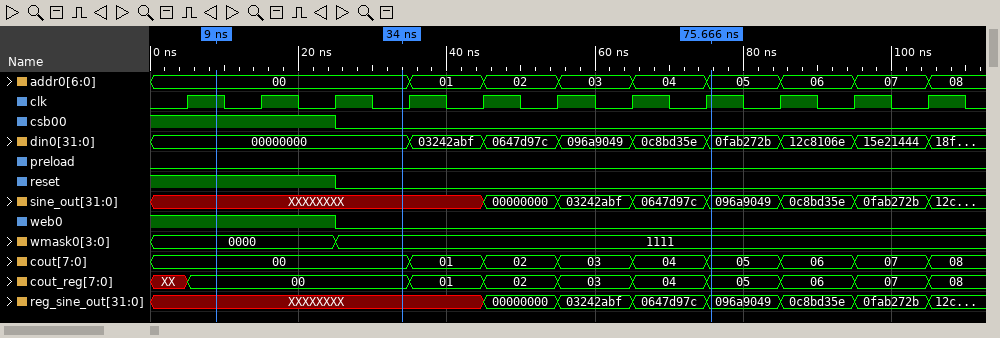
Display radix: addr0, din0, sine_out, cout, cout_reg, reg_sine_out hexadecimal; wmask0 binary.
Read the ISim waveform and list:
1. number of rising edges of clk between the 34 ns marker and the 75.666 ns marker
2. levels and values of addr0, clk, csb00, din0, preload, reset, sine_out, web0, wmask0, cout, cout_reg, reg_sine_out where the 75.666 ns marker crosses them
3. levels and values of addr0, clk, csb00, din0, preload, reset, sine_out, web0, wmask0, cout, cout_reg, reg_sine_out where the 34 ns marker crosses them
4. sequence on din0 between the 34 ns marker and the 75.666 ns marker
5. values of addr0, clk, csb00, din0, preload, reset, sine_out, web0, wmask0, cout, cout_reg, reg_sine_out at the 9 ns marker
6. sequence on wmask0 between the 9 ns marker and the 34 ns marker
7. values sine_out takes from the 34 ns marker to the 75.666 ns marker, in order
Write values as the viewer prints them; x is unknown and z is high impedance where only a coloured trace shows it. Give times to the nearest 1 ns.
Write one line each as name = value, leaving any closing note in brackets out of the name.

number of rising edges of clk between the 34 ns marker and the 75.666 ns marker = 5
levels and values of addr0, clk, csb00, din0, preload, reset, sine_out, web0, wmask0, cout, cout_reg, reg_sine_out where the 75.666 ns marker crosses them = addr0=05, clk=1, csb00=0, din0=0fab272b, preload=0, reset=0, sine_out=096a9049, web0=0, wmask0=1111, cout=05, cout_reg=05, reg_sine_out=096a9049
levels and values of addr0, clk, csb00, din0, preload, reset, sine_out, web0, wmask0, cout, cout_reg, reg_sine_out where the 34 ns marker crosses them = addr0=00, clk=0, csb00=0, din0=00000000, preload=0, reset=0, sine_out=XXXXXXXX, web0=0, wmask0=1111, cout=00, cout_reg=00, reg_sine_out=XXXXXXXX
sequence on din0 between the 34 ns marker and the 75.666 ns marker = 00000000, 03242abf, 0647d97c, 096a9049, 0c8bd35e, 0fab272b
values of addr0, clk, csb00, din0, preload, reset, sine_out, web0, wmask0, cout, cout_reg, reg_sine_out at the 9 ns marker = addr0=00, clk=1, csb00=1, din0=00000000, preload=0, reset=1, sine_out=XXXXXXXX, web0=1, wmask0=0000, cout=00, cout_reg=00, reg_sine_out=XXXXXXXX
sequence on wmask0 between the 9 ns marker and the 34 ns marker = 0000, 1111
values sine_out takes from the 34 ns marker to the 75.666 ns marker, in order = XXXXXXXX, 00000000, 03242abf, 0647d97c, 096a9049
